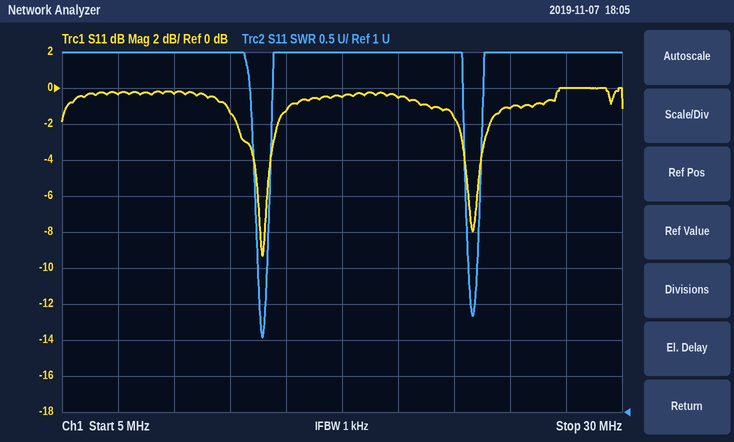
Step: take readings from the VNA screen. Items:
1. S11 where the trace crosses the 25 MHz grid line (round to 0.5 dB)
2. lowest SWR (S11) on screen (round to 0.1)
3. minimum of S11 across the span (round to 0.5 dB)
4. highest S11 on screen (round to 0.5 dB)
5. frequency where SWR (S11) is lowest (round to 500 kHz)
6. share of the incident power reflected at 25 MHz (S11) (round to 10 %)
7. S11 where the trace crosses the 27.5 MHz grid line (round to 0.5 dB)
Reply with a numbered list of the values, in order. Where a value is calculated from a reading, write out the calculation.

1. -1.0 dB
2. 2.0
3. -9.5 dB
4. 0.0 dB
5. 14.0 MHz
6. 10^(-1/10) ≈ 79.4 %, so 80 % to the nearest 10 %
7. 0.0 dB
